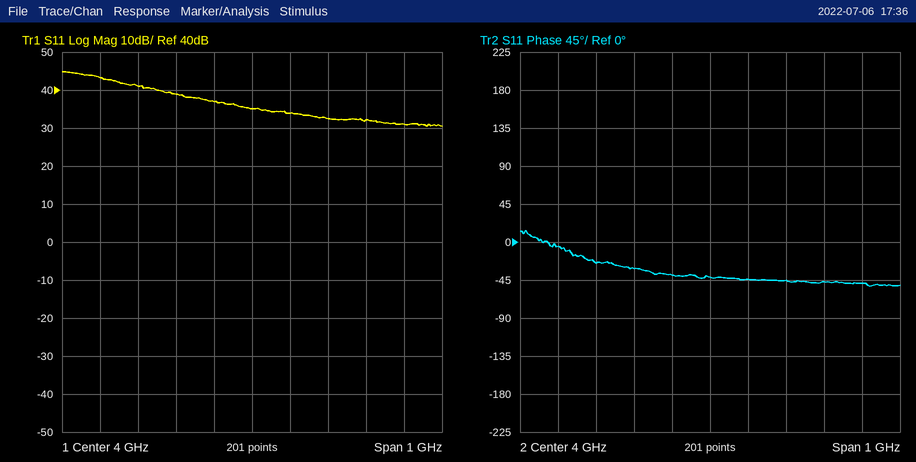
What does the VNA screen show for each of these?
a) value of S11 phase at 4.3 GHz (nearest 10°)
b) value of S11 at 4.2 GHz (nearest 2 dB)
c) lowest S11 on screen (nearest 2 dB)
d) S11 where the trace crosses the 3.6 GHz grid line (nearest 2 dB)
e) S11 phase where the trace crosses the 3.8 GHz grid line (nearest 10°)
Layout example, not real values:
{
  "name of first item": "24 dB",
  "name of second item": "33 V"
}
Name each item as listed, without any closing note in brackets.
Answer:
{
  "value of S11 phase at 4.3 GHz": "-50°",
  "value of S11 at 4.2 GHz": "32 dB",
  "lowest S11 on screen": "30 dB",
  "S11 where the trace crosses the 3.6 GHz grid line": "44 dB",
  "S11 phase where the trace crosses the 3.8 GHz grid line": "-30°"
}
